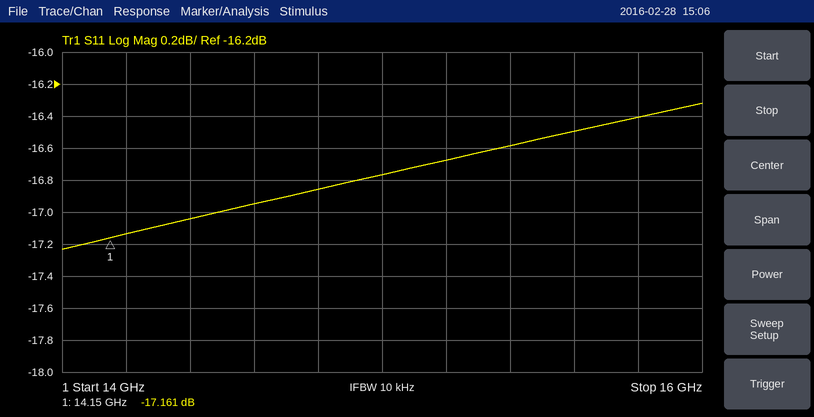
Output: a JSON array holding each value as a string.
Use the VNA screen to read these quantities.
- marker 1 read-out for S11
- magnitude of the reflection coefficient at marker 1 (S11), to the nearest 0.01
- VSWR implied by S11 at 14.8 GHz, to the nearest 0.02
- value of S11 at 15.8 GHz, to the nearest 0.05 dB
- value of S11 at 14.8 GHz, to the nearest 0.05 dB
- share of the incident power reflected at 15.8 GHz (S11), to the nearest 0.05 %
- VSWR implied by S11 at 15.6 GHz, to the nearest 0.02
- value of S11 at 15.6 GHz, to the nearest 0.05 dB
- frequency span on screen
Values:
["-17.161 dB", "0.14", "1.34", "-16.40 dB", "-16.85 dB", "2.30 %", "1.36", "-16.50 dB", "2 GHz"]
